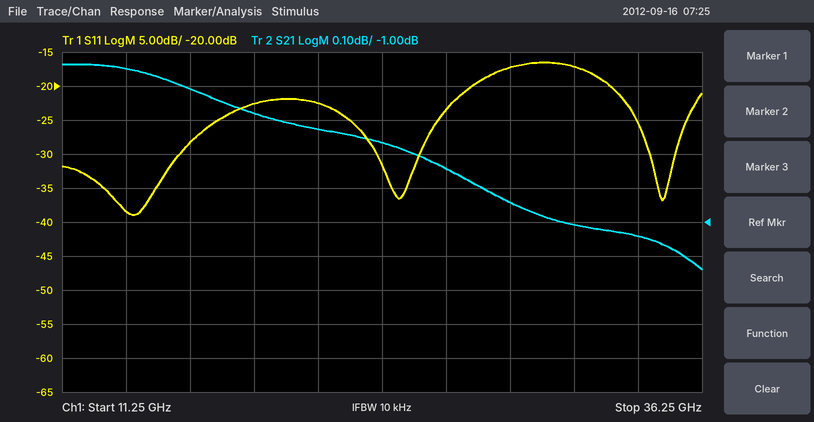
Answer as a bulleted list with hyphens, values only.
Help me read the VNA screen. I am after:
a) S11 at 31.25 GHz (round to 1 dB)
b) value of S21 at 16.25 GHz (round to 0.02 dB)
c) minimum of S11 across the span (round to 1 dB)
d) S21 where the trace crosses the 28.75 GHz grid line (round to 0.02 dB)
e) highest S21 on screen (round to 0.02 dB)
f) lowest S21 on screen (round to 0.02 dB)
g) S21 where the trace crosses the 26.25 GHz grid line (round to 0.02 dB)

- -17 dB
- -0.60 dB
- -39 dB
- -0.94 dB
- -0.54 dB
- -1.14 dB
- -0.84 dB
